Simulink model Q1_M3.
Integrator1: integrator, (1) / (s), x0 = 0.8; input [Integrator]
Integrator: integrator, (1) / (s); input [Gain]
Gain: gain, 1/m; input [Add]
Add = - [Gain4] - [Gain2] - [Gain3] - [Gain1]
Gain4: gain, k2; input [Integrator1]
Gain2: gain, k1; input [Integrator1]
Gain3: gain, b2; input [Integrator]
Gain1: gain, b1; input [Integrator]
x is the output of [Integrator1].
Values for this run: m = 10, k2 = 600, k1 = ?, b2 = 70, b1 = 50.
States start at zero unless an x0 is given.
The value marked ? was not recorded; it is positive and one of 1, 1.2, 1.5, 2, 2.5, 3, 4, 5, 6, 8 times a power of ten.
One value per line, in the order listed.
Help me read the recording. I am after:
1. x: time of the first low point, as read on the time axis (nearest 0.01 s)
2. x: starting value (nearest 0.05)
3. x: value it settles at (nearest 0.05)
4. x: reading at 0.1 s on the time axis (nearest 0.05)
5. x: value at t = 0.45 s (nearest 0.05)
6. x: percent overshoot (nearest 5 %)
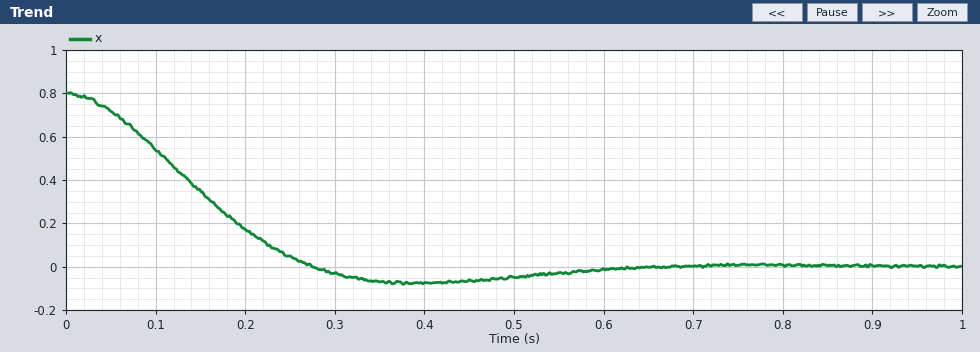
0.39 s
0.80
0.00
0.55
-0.05
10 %
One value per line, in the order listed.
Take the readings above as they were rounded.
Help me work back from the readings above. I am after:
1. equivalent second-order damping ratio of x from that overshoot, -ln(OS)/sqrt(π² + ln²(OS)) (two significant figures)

0.59
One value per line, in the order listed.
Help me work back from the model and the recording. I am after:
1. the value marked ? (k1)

400
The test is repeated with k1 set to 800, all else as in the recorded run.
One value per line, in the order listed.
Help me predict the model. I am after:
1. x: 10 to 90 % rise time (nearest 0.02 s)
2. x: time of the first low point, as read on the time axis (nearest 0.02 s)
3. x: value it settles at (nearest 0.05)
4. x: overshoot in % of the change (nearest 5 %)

0.14 s
0.30 s
0.00
15 %
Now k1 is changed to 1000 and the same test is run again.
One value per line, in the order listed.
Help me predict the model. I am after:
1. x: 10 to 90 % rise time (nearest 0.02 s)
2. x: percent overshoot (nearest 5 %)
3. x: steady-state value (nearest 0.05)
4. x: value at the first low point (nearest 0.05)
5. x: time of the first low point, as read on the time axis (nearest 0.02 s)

0.12 s
20 %
0.00
-0.15
0.28 s
